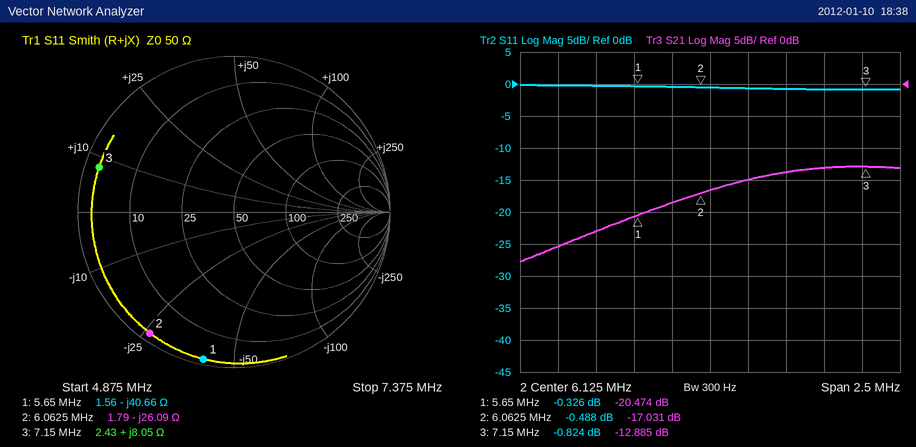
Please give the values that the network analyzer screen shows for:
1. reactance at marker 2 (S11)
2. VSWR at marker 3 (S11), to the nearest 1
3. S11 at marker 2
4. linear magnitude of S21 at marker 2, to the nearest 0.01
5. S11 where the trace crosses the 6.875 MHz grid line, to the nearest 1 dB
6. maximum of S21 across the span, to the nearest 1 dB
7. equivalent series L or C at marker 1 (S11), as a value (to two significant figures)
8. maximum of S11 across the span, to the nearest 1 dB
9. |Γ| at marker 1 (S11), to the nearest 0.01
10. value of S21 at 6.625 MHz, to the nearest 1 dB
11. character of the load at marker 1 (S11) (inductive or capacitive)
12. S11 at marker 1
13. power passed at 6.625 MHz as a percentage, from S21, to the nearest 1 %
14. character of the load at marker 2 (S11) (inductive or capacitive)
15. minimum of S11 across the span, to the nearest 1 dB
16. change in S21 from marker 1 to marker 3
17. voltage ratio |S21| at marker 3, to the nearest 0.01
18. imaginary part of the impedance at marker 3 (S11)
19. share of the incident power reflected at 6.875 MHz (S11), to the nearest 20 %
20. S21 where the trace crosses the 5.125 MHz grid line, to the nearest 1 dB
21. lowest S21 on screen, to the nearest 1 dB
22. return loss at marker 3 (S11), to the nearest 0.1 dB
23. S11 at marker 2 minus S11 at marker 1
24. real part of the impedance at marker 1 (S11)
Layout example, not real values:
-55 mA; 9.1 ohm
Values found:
-26.09 Ω; 21; -0.488 dB; 0.14; -1 dB; -13 dB; 690 pF; 0 dB; 0.96; -14 dB; capacitive; -0.326 dB; 4 %; capacitive; -1 dB; 7.589 dB; 0.23; +8.05 Ω; 80 %; -25 dB; -28 dB; 0.8 dB; -0.162 dB; 1.56 Ω
